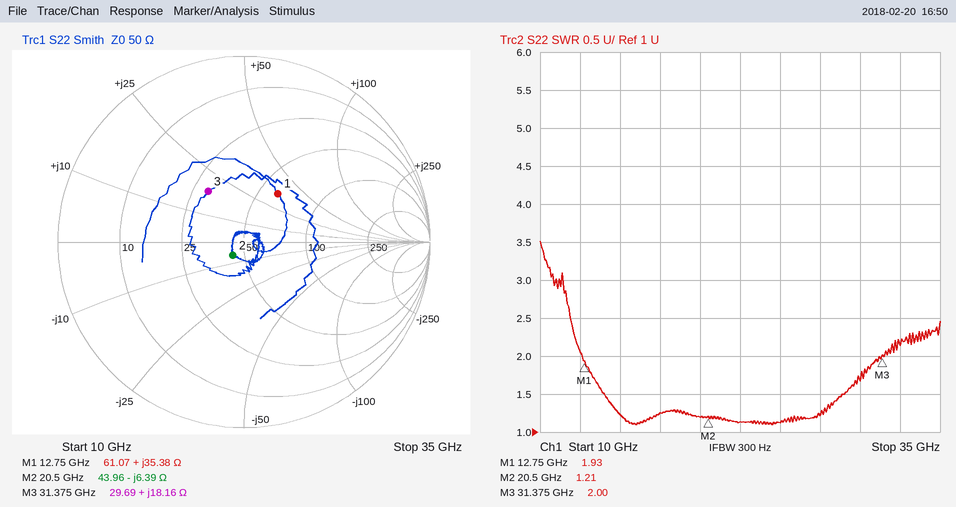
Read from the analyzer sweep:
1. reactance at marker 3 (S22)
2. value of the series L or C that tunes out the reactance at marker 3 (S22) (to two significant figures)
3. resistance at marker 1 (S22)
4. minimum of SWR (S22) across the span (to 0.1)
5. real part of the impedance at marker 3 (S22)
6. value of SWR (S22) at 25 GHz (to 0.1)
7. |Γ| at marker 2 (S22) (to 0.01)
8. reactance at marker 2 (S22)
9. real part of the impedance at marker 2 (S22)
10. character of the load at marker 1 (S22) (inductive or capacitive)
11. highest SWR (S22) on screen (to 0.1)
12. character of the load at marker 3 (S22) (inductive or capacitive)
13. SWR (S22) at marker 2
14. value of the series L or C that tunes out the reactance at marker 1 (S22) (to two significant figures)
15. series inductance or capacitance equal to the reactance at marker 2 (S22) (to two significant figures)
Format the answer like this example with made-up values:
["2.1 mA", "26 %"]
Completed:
["+18.16 Ω", "280 fF", "61.07 Ω", "1.1", "29.69 Ω", "1.1", "0.09", "-6.39 Ω", "43.96 Ω", "inductive", "3.5", "inductive", "1.21", "350 fF", "1.2 pF"]
